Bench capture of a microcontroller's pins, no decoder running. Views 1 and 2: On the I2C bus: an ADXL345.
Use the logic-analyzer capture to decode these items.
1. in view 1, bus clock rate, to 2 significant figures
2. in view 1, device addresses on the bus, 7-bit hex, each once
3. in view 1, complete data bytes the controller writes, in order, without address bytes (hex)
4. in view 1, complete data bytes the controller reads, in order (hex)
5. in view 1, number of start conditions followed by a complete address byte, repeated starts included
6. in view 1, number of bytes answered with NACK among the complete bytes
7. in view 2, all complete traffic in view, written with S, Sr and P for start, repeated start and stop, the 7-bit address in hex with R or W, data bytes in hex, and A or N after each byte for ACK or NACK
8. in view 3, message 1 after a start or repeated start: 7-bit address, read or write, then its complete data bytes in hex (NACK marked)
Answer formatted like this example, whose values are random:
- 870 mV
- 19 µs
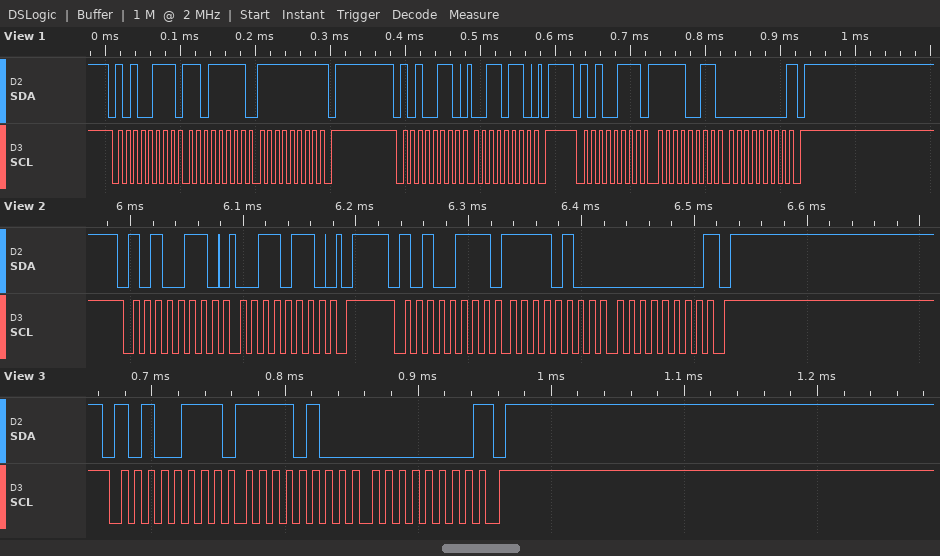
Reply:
- 100 kHz
- 0x53
- 36
- DF FF F3 00
- 3
- 2
- S 53W A 36 A P S 53R A F4 A 00 N P
- 0x53 read: F4 00 NACK
